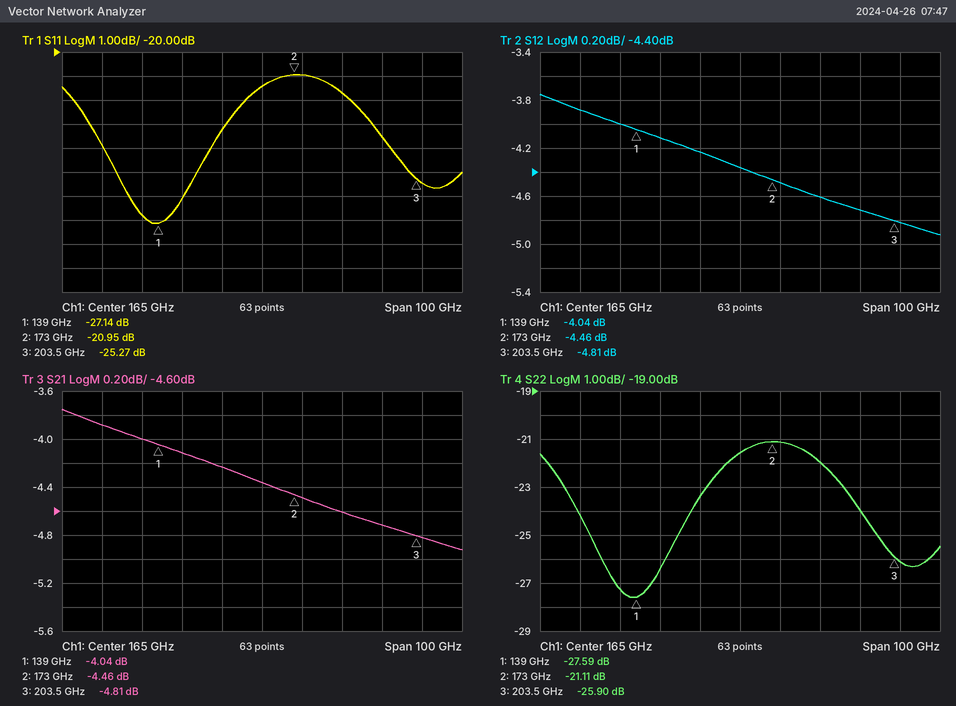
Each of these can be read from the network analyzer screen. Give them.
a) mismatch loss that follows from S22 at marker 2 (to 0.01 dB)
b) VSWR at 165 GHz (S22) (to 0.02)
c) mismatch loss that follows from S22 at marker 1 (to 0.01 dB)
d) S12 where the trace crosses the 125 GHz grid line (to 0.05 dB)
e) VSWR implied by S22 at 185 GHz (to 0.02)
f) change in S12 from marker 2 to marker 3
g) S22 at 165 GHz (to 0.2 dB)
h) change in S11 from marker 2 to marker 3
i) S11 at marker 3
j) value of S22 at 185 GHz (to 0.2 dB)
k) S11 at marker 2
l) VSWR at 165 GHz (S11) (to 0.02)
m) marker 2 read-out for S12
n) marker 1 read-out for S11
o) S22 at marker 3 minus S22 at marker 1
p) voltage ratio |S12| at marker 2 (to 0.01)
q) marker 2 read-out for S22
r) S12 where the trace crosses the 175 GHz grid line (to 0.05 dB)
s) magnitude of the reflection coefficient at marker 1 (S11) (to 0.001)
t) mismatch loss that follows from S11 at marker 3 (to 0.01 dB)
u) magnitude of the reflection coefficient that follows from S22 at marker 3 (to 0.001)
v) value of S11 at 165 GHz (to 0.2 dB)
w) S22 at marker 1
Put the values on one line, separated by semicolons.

0.03 dB; 1.18; 0.01 dB; -3.90 dB; 1.18; -0.35 dB; -21.6 dB; -4.32 dB; -25.27 dB; -22.0 dB; -20.95 dB; 1.18; -4.46 dB; -27.14 dB; 1.69 dB; 0.60; -21.11 dB; -4.50 dB; 0.044; 0.01 dB; 0.051; -21.4 dB; -27.59 dB
